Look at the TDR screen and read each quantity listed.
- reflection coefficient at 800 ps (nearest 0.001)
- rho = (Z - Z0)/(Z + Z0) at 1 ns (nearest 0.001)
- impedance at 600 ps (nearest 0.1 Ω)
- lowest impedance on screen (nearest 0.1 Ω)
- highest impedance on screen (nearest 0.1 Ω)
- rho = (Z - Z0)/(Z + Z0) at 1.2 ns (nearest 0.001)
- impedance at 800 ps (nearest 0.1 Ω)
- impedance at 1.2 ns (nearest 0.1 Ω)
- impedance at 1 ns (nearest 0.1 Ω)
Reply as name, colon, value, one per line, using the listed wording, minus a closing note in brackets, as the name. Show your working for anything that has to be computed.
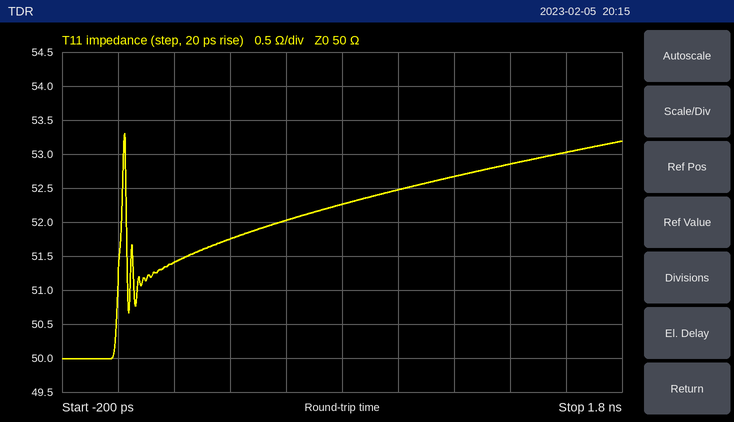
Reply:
reflection coefficient at 800 ps: (52.3 − 50)/(52.3 + 50) ≈ +0.022
rho = (Z - Z0)/(Z + Z0) at 1 ns: (52.5 − 50)/(52.5 + 50) ≈ +0.024
impedance at 600 ps: 52.0 Ω
lowest impedance on screen: 50.0 Ω
highest impedance on screen: 53.3 Ω
rho = (Z - Z0)/(Z + Z0) at 1.2 ns: (52.7 − 50)/(52.7 + 50) ≈ +0.026
impedance at 800 ps: 52.3 Ω
impedance at 1.2 ns: 52.7 Ω
impedance at 1 ns: 52.5 Ω
